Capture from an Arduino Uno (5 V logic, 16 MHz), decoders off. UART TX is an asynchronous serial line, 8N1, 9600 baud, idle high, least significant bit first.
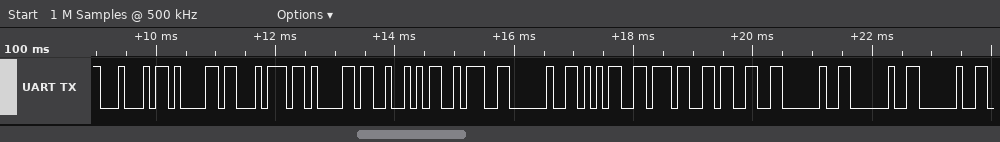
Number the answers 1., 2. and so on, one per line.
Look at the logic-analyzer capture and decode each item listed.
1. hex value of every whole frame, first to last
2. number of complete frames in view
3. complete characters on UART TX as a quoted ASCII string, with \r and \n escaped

1. 44 61 74 61 52 3A 20 35 37 33 20 20 20
2. 13
3. "DataR: 573   "
